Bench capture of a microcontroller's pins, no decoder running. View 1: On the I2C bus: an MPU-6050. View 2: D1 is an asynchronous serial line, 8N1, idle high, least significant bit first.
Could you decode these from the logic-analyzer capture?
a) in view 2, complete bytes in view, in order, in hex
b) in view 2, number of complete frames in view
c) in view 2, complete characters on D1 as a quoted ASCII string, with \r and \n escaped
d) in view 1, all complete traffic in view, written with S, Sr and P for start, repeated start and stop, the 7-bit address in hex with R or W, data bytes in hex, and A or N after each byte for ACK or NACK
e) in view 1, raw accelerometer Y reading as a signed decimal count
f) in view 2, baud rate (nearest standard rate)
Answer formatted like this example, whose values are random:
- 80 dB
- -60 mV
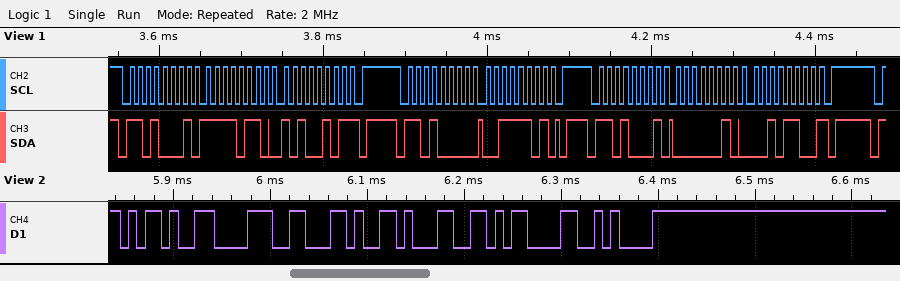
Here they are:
- 2D 38 2C 31 0D 0A
- 6
- "-8,1\r\n"
- S 68R A F6 A A5 N P S 68W A 3D A P S 68R A 02 A 2C N P
- 556
- 115200 baud
